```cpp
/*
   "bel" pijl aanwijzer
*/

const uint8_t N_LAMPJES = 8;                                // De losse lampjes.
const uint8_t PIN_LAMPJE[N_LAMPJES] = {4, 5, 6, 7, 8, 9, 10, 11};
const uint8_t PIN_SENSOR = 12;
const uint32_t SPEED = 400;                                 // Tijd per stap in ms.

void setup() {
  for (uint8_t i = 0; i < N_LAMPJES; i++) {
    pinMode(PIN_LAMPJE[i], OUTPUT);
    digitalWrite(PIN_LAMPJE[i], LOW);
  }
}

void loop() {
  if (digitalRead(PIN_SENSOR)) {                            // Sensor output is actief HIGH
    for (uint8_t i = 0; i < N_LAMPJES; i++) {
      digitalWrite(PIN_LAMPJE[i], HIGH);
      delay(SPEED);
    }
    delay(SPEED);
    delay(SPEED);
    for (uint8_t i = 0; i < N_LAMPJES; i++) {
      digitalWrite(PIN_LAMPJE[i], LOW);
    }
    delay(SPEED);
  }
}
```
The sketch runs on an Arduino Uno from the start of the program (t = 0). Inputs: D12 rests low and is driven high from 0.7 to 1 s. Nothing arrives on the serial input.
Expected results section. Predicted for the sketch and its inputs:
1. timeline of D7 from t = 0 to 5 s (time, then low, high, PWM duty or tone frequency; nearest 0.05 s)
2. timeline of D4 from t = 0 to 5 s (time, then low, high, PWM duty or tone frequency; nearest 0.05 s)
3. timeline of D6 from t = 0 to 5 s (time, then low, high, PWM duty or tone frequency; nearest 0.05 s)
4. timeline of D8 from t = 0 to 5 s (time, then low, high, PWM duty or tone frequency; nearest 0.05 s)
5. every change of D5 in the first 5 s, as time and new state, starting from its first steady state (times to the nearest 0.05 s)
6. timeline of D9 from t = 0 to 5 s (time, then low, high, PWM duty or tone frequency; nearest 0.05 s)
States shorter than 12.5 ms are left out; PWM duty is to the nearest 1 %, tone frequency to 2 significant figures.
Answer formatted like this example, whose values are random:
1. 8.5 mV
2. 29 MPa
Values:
1. 0 s low; 1.9 s high; 4.7 s low
2. 0 s low; 0.7 s high; 4.7 s low
3. 0 s low; 1.5 s high; 4.7 s low
4. 0 s low; 2.3 s high; 4.7 s low
5. 0 s low; 1.1 s high; 4.7 s low
6. 0 s low; 2.7 s high; 4.7 s low
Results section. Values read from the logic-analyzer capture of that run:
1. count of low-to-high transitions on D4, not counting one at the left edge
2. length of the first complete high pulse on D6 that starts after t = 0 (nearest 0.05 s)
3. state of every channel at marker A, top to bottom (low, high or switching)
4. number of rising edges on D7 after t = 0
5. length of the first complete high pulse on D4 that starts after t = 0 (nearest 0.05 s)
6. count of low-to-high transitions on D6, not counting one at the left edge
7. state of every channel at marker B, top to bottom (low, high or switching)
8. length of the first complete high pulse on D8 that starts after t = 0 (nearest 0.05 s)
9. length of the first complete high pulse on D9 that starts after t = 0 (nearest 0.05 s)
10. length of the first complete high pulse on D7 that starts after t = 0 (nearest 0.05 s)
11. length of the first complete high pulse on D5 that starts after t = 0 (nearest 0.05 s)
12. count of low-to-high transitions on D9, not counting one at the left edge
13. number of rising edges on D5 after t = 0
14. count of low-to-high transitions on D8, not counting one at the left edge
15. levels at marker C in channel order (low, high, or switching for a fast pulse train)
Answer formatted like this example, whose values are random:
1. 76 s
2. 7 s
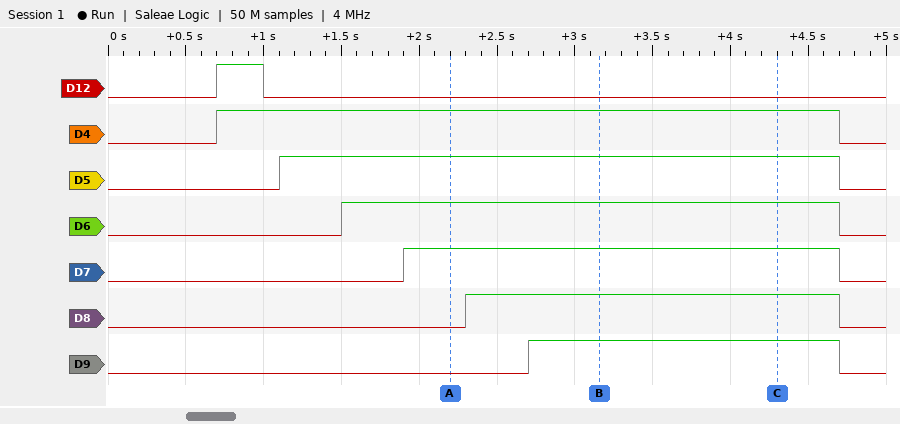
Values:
1. 1
2. 3.20 s
3. D12 low, D4 high, D5 high, D6 high, D7 high, D8 low, D9 low
4. 1
5. 4.00 s
6. 1
7. D12 low, D4 high, D5 high, D6 high, D7 high, D8 high, D9 high
8. 2.40 s
9. 2.00 s
10. 2.80 s
11. 3.60 s
12. 1
13. 1
14. 1
15. D12 low, D4 high, D5 high, D6 high, D7 high, D8 high, D9 high
